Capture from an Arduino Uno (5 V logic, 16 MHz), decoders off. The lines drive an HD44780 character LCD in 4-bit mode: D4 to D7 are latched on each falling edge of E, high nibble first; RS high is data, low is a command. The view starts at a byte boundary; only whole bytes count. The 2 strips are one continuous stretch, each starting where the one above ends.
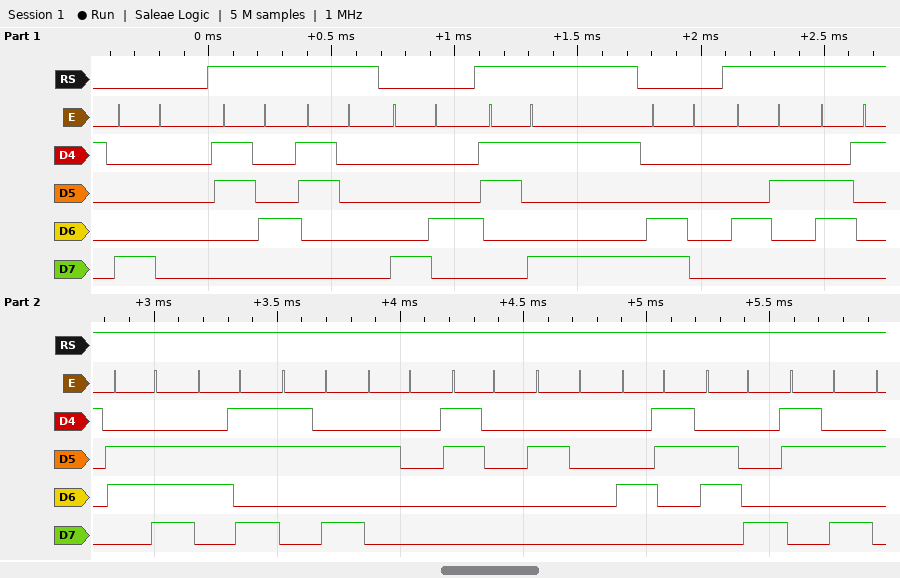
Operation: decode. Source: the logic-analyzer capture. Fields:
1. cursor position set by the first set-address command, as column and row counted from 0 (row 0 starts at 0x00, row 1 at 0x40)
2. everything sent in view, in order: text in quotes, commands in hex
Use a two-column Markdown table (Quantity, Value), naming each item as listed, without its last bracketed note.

| Quantity | Value |
|---|---|
| cursor position set by the first set-address command, as column and row counted from 0 | column 0, row 0 |
| everything sent in view, in order: text in quotes, commands in hex | 0x80 "40" 0x84 "9" 0xC0 "Bank: 0 Ch:" |
